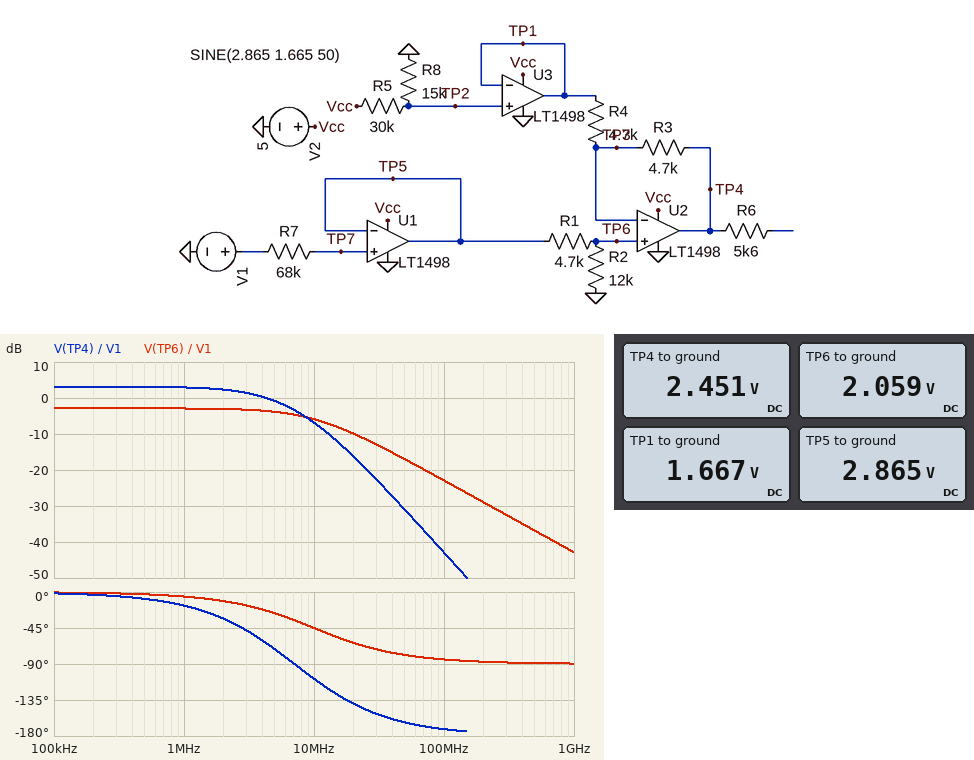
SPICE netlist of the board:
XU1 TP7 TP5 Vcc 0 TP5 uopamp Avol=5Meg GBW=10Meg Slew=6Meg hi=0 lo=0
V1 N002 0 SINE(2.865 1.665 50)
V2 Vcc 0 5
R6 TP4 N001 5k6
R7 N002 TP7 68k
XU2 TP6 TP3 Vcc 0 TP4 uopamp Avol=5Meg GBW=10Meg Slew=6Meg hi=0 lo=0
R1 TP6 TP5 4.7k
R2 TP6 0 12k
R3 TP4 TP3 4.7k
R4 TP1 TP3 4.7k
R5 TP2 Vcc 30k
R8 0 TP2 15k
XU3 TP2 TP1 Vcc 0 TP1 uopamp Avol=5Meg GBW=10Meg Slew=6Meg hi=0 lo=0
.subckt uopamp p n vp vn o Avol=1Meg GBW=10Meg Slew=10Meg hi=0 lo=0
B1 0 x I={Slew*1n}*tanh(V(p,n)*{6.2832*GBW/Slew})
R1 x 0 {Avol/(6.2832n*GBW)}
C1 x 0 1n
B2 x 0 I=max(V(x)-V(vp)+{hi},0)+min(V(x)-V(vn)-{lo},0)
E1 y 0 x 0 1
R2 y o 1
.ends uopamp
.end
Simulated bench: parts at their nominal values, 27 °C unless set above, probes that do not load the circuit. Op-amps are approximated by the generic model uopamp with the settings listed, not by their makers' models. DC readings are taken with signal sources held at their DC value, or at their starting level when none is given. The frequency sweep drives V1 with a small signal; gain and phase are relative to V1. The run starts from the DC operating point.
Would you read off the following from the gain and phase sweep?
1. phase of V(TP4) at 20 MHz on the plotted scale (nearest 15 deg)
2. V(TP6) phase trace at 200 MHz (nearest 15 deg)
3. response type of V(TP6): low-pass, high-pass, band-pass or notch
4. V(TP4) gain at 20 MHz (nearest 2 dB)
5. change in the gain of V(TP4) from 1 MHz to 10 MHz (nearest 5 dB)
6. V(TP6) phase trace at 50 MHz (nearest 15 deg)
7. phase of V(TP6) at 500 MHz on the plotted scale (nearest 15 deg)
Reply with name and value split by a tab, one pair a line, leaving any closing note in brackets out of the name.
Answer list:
phase of V(TP4) at 20 MHz on the plotted scale	-135 deg
V(TP6) phase trace at 200 MHz	-90 deg
response type of V(TP6): low-pass, high-pass, band-pass or notch	low-pass
V(TP4) gain at 20 MHz	-16 dB
change in the gain of V(TP4) from 1 MHz to 10 MHz	-10 dB
V(TP6) phase trace at 50 MHz	-75 deg
phase of V(TP6) at 500 MHz on the plotted scale	-90 deg
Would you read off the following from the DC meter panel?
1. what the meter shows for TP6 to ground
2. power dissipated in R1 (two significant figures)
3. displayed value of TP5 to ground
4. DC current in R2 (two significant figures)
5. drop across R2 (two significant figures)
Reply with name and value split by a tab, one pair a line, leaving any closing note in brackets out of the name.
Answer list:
what the meter shows for TP6 to ground	2.059 V
power dissipated in R1	140 µW
displayed value of TP5 to ground	2.865 V
DC current in R2	170 µA
drop across R2	2.1 V
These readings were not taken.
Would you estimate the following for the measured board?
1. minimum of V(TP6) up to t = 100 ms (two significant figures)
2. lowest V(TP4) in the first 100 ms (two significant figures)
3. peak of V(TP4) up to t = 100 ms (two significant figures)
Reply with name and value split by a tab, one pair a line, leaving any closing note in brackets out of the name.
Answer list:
minimum of V(TP6) up to t = 100 ms	860 mV
lowest V(TP4) in the first 100 ms	58 mV
peak of V(TP4) up to t = 100 ms	4.8 V
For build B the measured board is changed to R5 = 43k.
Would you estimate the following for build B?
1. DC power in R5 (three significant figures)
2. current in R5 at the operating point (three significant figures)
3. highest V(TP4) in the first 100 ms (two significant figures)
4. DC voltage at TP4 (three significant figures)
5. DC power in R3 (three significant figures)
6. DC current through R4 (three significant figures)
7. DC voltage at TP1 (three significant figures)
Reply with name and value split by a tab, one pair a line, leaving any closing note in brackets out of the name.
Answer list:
DC power in R5	320 µW
current in R5 at the operating point	86.2 µA
highest V(TP4) in the first 100 ms	5.0 V
DC voltage at TP4	2.82 V
DC power in R3	125 µW
DC current through R4	163 µA
DC voltage at TP1	1.29 V
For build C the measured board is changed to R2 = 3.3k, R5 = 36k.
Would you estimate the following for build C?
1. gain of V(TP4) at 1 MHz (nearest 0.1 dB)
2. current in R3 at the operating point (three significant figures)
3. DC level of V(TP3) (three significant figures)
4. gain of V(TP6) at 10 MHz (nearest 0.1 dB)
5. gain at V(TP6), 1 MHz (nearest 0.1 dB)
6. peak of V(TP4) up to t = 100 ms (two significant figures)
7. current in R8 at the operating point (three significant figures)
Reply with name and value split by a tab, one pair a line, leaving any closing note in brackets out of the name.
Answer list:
gain of V(TP4) at 1 MHz	-1.9 dB
current in R3 at the operating point	61.4 µA
DC level of V(TP3)	1.18 V
gain of V(TP6) at 10 MHz	-10.7 dB
gain at V(TP6), 1 MHz	-7.7 dB
peak of V(TP4) up to t = 100 ms	2.3 V
current in R8 at the operating point	98.0 µA
